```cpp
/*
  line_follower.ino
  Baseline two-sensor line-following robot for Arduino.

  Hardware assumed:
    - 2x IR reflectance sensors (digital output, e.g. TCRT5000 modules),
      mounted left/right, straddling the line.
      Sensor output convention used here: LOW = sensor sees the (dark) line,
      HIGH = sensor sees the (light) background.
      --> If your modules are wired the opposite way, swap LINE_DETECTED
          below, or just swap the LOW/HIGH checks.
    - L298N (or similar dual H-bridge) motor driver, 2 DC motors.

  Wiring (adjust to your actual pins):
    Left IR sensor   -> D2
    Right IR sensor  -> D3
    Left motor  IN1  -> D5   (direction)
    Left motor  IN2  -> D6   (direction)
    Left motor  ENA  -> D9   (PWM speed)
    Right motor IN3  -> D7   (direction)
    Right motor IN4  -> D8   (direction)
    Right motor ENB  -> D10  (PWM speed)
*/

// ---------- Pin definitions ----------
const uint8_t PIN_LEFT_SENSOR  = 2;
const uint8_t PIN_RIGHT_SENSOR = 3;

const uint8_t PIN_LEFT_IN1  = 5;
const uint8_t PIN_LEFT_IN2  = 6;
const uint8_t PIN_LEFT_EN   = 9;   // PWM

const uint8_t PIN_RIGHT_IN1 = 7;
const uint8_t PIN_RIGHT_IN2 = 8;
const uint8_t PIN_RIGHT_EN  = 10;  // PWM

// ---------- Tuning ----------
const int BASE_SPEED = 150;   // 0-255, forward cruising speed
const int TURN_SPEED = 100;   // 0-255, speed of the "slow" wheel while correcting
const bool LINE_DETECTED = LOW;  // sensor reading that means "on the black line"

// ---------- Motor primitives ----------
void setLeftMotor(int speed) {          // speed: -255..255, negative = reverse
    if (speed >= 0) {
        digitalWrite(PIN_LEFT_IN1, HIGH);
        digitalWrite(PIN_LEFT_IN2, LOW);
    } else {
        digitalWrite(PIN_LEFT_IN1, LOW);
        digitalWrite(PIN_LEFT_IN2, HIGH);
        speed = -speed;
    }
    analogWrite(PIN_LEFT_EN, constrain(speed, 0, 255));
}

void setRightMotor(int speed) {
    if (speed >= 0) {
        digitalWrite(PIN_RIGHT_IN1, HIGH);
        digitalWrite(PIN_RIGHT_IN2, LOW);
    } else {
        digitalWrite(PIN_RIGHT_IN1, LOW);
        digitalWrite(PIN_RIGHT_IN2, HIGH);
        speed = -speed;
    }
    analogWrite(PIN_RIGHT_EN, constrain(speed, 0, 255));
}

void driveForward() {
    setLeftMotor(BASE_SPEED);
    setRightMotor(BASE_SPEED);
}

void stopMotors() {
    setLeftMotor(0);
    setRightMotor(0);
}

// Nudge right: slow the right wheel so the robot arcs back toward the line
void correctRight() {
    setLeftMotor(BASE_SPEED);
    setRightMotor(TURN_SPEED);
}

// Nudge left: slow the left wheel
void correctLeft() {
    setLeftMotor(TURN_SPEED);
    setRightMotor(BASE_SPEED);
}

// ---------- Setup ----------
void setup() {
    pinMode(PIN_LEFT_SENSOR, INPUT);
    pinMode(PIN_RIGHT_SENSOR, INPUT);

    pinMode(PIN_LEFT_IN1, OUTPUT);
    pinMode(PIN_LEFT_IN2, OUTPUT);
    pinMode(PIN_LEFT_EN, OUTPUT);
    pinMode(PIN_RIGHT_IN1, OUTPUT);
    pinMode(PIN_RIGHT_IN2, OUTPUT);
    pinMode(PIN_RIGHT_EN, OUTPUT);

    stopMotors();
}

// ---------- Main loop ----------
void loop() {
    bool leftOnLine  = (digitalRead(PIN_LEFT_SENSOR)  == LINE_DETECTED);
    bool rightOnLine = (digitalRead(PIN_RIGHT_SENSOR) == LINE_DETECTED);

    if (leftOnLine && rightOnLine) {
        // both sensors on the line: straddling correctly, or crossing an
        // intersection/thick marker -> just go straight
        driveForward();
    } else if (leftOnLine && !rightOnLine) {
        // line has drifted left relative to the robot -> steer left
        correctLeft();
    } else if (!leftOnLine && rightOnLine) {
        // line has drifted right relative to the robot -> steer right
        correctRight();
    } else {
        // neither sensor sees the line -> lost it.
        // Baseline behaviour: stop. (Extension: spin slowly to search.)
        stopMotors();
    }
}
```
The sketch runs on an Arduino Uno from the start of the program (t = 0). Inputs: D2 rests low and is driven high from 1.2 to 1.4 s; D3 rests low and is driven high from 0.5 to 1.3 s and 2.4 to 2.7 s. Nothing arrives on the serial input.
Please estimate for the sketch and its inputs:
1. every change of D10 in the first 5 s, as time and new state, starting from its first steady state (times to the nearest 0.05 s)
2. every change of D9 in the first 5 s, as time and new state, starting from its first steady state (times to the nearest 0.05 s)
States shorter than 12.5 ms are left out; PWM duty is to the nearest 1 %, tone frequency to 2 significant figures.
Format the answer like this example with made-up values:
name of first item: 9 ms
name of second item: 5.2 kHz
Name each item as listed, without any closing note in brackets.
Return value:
every change of D10 in the first 5 s, as time and new state, starting from its first steady state: 0 s PWM 59 %; 1.2 s low; 1.3 s PWM 39 %; 1.4 s PWM 59 %
every change of D9 in the first 5 s, as time and new state, starting from its first steady state: 0 s PWM 59 %; 0.5 s PWM 39 %; 1.2 s low; 1.3 s PWM 59 %; 2.4 s PWM 39 %; 2.7 s PWM 59 %
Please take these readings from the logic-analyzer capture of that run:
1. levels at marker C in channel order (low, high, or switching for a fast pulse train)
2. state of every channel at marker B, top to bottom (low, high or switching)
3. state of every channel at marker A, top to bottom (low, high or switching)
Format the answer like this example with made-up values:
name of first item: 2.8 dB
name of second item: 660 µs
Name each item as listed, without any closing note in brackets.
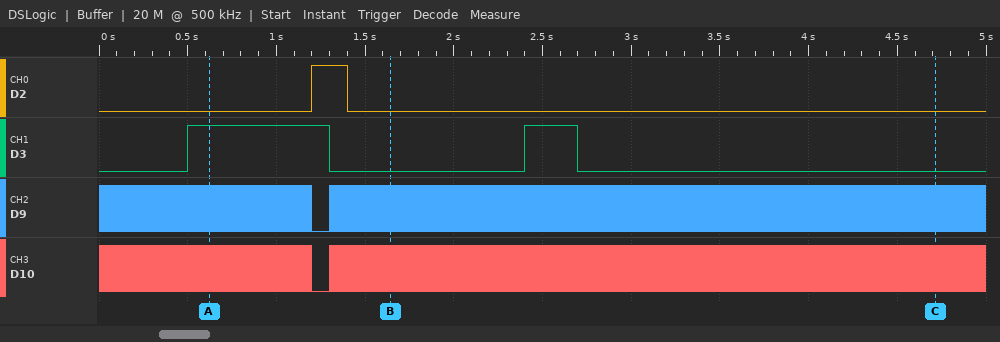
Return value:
levels at marker C in channel order: D2 low, D3 low, D9 switching, D10 switching
state of every channel at marker B, top to bottom: D2 low, D3 low, D9 switching, D10 switching
state of every channel at marker A, top to bottom: D2 low, D3 high, D9 switching, D10 switching
